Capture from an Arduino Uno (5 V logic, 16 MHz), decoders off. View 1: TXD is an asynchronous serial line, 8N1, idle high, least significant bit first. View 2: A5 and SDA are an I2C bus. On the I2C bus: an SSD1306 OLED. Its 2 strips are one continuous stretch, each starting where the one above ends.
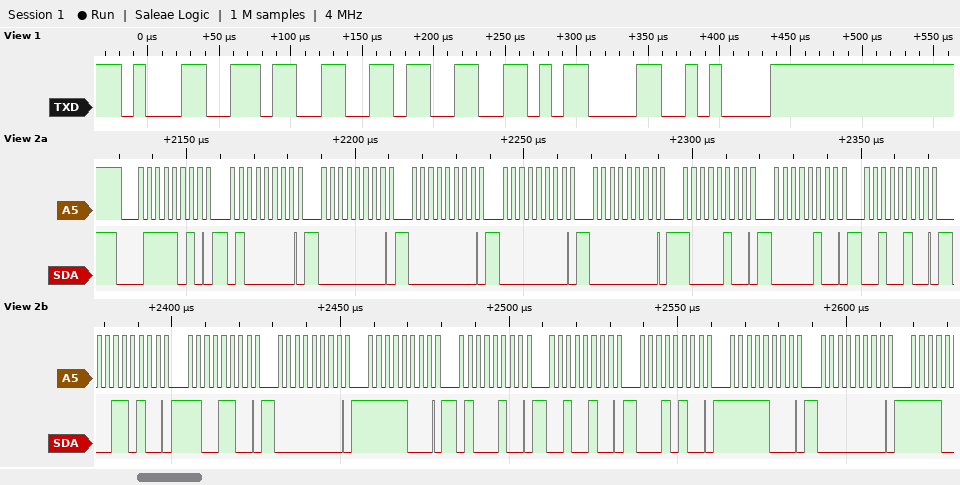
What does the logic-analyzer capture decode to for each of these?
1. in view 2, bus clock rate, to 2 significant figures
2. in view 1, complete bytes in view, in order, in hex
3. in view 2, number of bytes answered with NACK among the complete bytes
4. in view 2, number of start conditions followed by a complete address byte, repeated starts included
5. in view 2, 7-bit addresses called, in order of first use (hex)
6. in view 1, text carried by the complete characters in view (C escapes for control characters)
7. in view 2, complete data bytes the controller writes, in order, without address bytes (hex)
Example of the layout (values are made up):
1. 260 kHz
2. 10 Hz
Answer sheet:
1. 400 kHz
2. 31 33 33 0D 0A
3. 0
4. 1
5. 0x3D
6. "133\r\n"
7. 40 00 00 00 00 84 04 24 34 CC 00 F8 44 24 14 F8 00
